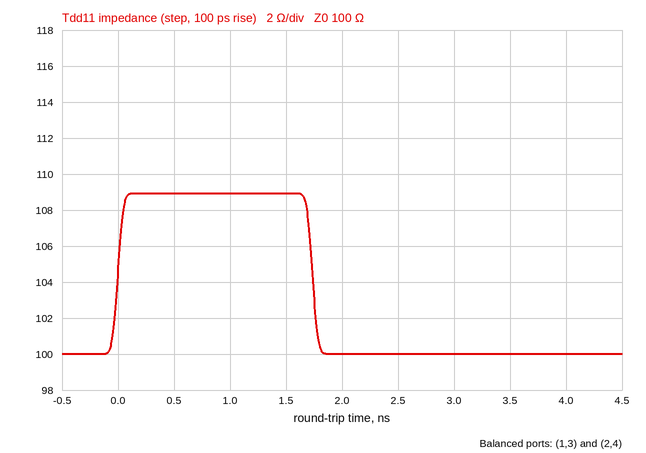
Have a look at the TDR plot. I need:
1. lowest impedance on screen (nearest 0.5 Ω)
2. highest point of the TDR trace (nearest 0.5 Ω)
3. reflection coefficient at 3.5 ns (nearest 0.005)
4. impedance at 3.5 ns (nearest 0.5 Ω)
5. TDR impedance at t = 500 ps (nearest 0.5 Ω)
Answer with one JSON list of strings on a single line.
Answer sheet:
["100.0 Ω", "109.0 Ω", "0.000", "100.0 Ω", "109.0 Ω"]
